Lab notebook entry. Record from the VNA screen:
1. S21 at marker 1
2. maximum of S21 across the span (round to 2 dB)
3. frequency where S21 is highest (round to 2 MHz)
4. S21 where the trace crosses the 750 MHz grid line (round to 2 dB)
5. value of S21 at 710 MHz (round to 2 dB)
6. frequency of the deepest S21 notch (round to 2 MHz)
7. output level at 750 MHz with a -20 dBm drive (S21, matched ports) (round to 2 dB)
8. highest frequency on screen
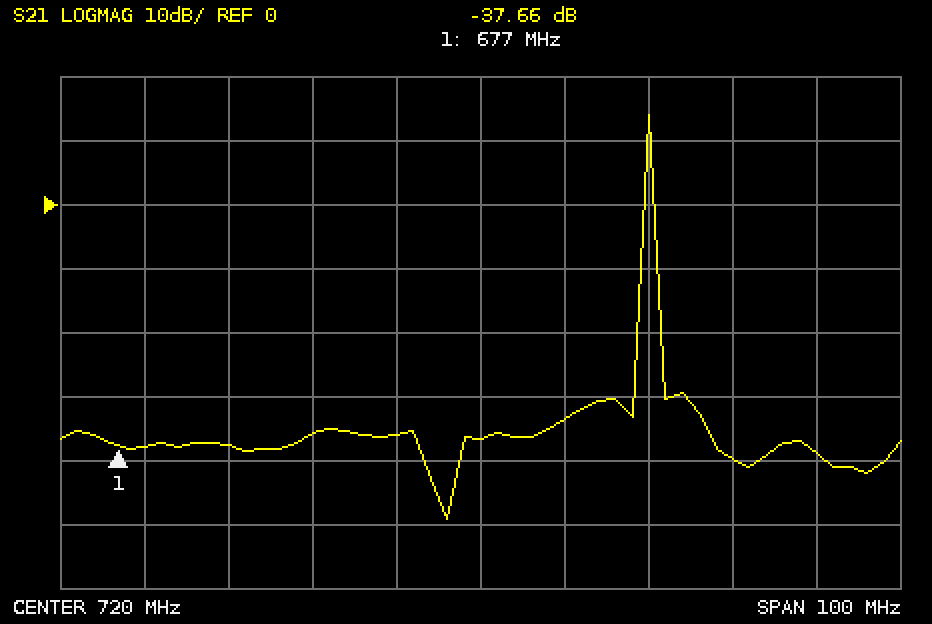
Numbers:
-37.66 dB
14 dB
740 MHz
-40 dB
-36 dB
716 MHz
-60 dBm
770 MHz
